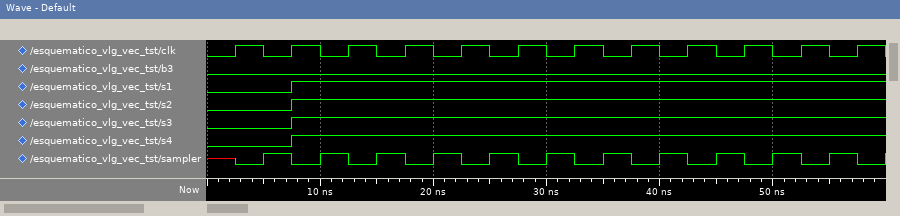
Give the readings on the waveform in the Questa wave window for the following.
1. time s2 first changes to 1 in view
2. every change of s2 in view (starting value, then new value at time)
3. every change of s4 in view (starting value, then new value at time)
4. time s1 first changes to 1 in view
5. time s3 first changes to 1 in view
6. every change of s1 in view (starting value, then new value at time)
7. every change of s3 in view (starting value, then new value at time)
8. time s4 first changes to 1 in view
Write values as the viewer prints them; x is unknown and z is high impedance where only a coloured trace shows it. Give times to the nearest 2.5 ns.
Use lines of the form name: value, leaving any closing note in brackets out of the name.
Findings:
time s2 first changes to 1 in view: 7.5 ns
every change of s2 in view: 0, 1 at 7.5 ns
every change of s4 in view: 0, 1 at 7.5 ns
time s1 first changes to 1 in view: 7.5 ns
time s3 first changes to 1 in view: 7.5 ns
every change of s1 in view: 0, 1 at 7.5 ns
every change of s3 in view: 0, 1 at 7.5 ns
time s4 first changes to 1 in view: 7.5 ns
